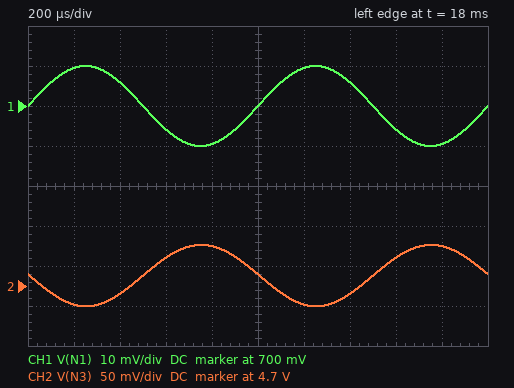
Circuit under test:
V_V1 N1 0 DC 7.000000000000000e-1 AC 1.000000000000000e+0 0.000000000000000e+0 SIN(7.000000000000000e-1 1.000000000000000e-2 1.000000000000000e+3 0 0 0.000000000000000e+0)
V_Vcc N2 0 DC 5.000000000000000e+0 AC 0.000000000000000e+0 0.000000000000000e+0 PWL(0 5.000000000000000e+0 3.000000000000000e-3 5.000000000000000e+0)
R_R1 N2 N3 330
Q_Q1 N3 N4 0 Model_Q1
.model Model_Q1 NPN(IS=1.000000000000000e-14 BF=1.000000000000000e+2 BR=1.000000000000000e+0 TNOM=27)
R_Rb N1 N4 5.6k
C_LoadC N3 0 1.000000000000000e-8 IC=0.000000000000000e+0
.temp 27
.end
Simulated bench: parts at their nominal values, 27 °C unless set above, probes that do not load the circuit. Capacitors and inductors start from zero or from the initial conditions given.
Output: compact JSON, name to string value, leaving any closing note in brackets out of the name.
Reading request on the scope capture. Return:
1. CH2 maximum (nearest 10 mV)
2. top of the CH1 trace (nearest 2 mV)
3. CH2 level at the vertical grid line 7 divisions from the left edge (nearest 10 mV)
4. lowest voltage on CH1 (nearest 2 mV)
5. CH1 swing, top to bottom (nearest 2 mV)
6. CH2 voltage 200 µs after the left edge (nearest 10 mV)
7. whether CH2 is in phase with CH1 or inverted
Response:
{"CH2 maximum": "4.75 V", "top of the CH1 trace": "710 mV", "CH2 level at the vertical grid line 7 divisions from the left edge": "4.69 V", "lowest voltage on CH1": "690 mV", "CH1 swing, top to bottom": "20 mV", "CH2 voltage 200 µs after the left edge": "4.68 V", "whether CH2 is in phase with CH1 or inverted": "inverted"}
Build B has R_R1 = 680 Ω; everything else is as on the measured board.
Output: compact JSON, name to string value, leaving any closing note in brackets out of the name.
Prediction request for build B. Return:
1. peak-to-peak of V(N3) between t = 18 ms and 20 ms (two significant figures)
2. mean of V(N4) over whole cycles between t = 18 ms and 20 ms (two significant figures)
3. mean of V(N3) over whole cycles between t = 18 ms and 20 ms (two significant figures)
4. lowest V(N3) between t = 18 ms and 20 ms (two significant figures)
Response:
{"peak-to-peak of V(N3) between t = 18 ms and 20 ms": "160 mV", "mean of V(N4) over whole cycles between t = 18 ms and 20 ms": "650 mV", "mean of V(N3) over whole cycles between t = 18 ms and 20 ms": "4.4 V", "lowest V(N3) between t = 18 ms and 20 ms": "4.3 V"}
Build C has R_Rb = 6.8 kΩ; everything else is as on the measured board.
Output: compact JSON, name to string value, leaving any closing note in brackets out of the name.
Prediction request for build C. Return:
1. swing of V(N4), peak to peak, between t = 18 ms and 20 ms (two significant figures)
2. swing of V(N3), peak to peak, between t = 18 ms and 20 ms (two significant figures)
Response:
{"swing of V(N4), peak to peak, between t = 18 ms and 20 ms": "6.7 mV", "swing of V(N3), peak to peak, between t = 18 ms and 20 ms": "65 mV"}
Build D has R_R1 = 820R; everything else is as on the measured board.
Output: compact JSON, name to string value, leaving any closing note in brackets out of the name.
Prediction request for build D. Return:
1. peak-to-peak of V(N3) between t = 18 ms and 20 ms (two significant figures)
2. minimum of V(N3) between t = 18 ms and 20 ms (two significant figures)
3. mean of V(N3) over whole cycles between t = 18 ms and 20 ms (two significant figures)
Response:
{"peak-to-peak of V(N3) between t = 18 ms and 20 ms": "190 mV", "minimum of V(N3) between t = 18 ms and 20 ms": "4.2 V", "mean of V(N3) over whole cycles between t = 18 ms and 20 ms": "4.3 V"}
